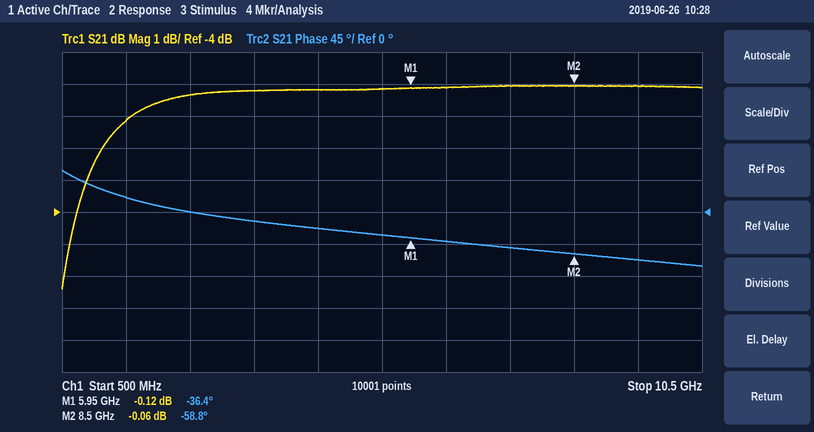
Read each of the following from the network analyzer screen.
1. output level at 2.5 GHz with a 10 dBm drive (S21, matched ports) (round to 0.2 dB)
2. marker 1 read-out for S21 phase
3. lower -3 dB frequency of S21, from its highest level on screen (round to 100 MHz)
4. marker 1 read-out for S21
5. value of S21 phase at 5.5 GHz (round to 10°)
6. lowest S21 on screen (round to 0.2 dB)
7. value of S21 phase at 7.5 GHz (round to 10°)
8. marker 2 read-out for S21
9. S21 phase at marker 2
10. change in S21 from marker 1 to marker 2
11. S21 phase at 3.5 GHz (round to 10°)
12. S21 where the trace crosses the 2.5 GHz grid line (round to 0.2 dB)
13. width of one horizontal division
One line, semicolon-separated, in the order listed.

9.6 dBm; -36.4°; 900 MHz; -0.12 dB; -30°; -6.4 dB; -50°; -0.06 dB; -58.8°; 0.06 dB; -10°; -0.4 dB; 1 GHz
